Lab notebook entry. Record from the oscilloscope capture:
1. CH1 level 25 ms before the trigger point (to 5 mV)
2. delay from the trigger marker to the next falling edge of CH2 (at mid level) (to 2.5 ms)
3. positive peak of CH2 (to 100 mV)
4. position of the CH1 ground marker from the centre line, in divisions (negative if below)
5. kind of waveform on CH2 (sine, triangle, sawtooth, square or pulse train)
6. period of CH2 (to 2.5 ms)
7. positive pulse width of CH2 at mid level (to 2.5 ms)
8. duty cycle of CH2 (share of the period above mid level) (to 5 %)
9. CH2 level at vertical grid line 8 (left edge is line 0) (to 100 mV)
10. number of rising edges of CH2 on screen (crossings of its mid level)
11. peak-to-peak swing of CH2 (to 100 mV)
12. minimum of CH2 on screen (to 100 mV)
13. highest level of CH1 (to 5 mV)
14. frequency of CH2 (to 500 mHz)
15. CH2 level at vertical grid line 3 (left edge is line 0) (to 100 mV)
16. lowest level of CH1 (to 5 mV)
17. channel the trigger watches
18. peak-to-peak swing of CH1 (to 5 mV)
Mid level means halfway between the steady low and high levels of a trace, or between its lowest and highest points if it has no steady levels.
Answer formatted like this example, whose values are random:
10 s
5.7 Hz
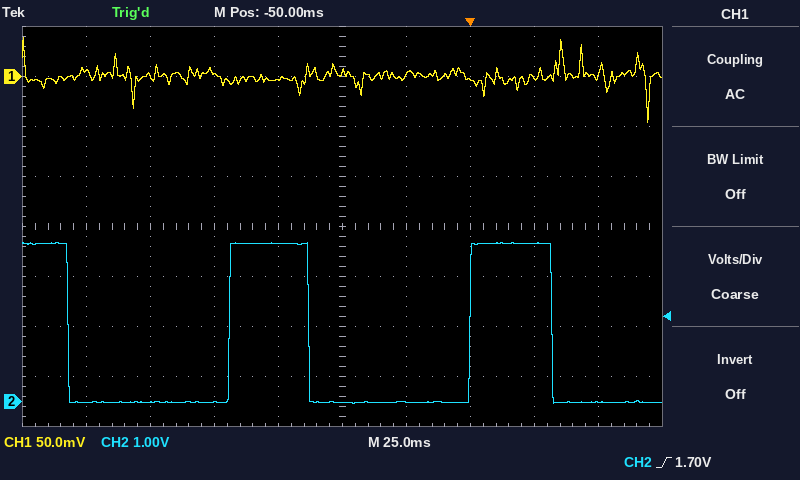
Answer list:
0 mV
32.5 ms
3.2 V
+3.0 div
pulse train
95.0 ms
32.5 ms
35 %
3.2 V
2
3.2 V
0.0 V
40 mV
10.5 Hz
0.0 V
-45 mV
CH2
85 mV
